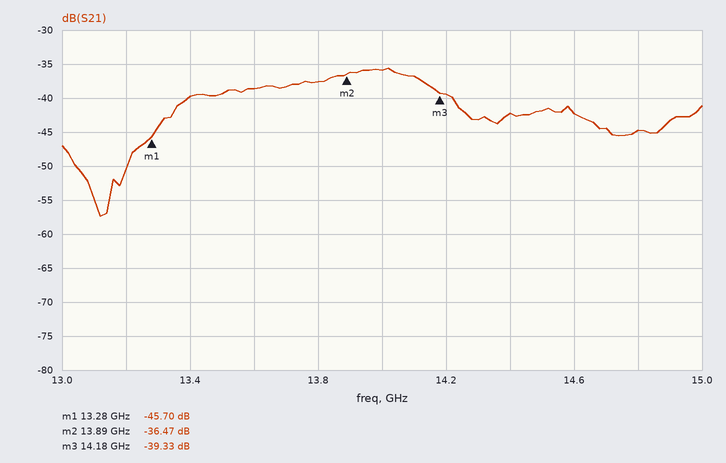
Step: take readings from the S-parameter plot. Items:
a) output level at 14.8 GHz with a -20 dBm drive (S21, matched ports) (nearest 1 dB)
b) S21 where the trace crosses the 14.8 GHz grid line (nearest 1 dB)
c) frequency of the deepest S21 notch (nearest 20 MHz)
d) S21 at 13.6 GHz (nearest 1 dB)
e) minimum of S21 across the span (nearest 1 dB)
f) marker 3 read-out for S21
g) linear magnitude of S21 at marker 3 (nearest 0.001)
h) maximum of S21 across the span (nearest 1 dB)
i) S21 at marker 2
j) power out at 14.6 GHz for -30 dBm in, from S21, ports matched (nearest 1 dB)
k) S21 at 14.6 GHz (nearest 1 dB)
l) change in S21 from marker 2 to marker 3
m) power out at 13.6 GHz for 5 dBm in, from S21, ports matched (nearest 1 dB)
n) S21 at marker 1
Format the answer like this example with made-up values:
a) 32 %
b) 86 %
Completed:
a) -65 dBm
b) -45 dB
c) 13.12 GHz
d) -39 dB
e) -57 dB
f) -39.33 dB
g) 0.011
h) -36 dB
i) -36.47 dB
j) -72 dBm
k) -42 dB
l) -2.86 dB
m) -34 dBm
n) -45.70 dB
